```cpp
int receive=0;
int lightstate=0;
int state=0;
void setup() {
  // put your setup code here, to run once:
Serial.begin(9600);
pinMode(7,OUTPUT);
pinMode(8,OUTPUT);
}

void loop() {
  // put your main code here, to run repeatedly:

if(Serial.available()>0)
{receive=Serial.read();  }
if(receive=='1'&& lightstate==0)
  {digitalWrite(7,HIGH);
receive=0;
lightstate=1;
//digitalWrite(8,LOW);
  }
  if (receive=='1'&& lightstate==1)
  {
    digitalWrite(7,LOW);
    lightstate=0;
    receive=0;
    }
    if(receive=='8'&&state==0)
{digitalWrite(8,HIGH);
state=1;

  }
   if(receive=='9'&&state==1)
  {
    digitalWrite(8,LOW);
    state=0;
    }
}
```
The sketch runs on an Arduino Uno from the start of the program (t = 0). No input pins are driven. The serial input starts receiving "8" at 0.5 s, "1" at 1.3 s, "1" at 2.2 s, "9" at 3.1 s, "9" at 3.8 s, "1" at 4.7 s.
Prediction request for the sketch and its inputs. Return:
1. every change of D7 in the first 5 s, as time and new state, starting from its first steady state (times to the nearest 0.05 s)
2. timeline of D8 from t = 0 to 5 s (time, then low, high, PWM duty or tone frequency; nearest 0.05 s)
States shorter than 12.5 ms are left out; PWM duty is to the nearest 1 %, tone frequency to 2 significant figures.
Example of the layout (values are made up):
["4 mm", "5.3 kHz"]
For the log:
["0 s low; 1.3 s high; 2.2 s low; 4.7 s high", "0 s low; 0.5 s high; 3.1 s low"]
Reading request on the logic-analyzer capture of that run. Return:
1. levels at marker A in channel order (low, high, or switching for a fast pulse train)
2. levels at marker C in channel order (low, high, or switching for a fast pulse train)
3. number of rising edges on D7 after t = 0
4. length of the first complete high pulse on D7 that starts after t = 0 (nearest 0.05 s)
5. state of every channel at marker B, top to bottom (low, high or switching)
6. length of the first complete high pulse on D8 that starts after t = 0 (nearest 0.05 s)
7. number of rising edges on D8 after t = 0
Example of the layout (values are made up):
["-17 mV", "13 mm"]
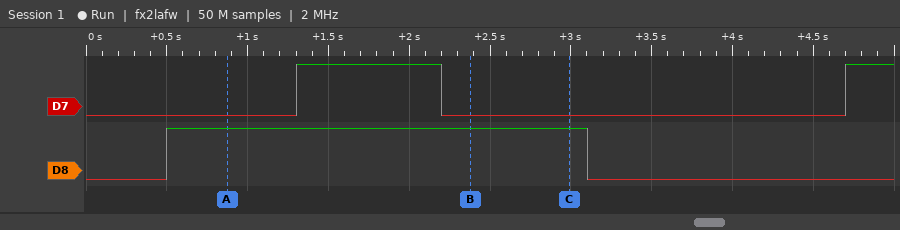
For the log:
["D7 low, D8 high", "D7 low, D8 high", "2", "0.90 s", "D7 low, D8 high", "2.60 s", "1"]
